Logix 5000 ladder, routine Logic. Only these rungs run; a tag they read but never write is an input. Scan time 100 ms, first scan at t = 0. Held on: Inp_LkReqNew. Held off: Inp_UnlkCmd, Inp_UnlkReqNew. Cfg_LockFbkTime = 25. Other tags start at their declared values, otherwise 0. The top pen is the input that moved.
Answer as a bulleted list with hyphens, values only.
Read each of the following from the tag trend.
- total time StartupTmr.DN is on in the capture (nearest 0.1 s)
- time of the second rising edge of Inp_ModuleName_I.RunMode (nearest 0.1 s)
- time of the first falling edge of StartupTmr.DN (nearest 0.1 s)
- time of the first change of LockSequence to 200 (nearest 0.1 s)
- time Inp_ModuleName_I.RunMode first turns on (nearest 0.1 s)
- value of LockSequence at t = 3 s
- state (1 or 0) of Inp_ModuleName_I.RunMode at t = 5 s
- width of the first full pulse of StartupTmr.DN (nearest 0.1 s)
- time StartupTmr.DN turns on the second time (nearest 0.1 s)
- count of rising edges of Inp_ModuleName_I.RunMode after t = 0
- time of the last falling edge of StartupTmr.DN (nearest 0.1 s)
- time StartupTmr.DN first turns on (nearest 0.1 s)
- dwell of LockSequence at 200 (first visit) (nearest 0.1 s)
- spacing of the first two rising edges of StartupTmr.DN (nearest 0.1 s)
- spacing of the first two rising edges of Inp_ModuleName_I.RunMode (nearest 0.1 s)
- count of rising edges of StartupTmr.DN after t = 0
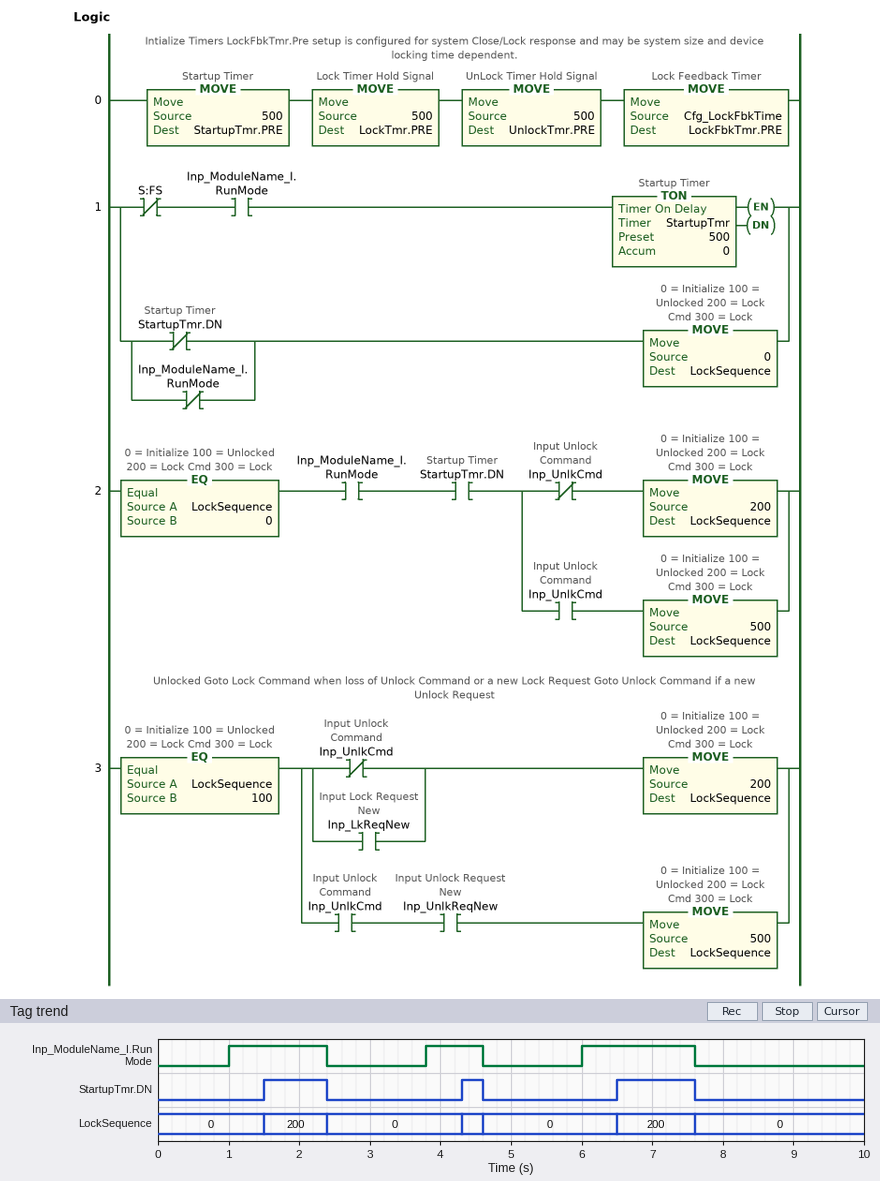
- 2.3 s
- 3.8 s
- 2.4 s
- 1.5 s
- 1.0 s
- 0
- 0
- 0.9 s
- 4.3 s
- 3
- 7.6 s
- 1.5 s
- 0.9 s
- 2.8 s
- 2.8 s
- 3
